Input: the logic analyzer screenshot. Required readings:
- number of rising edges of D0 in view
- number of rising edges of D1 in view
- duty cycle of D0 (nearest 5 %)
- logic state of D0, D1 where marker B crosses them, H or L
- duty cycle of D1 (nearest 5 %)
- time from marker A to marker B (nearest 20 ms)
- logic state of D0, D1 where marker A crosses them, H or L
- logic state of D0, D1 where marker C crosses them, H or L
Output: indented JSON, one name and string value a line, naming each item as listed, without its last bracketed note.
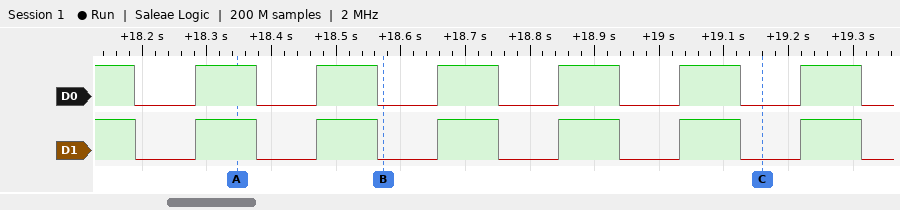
{
  "number of rising edges of D0 in view": "6",
  "number of rising edges of D1 in view": "6",
  "duty cycle of D0": "50 %",
  "logic state of D0, D1 where marker B crosses them, H or L": "D0=L, D1=L",
  "duty cycle of D1": "50 %",
  "time from marker A to marker B": "220 ms",
  "logic state of D0, D1 where marker A crosses them, H or L": "D0=H, D1=H",
  "logic state of D0, D1 where marker C crosses them, H or L": "D0=L, D1=L"
}
